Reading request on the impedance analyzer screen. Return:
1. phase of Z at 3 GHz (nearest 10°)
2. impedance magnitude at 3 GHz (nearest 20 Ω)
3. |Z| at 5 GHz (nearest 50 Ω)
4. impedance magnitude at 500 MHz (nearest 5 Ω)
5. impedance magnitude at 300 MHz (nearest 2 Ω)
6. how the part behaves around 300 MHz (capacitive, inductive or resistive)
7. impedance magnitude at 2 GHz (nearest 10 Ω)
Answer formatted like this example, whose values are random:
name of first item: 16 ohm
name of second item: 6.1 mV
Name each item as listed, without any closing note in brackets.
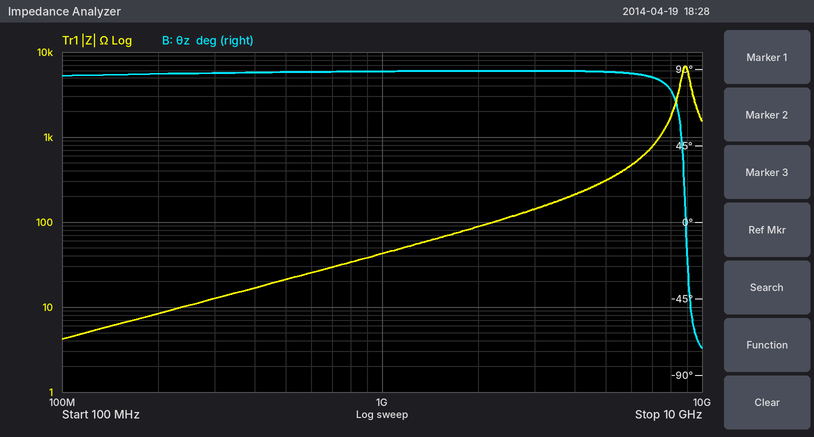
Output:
phase of Z at 3 GHz: 90°
impedance magnitude at 3 GHz: 140 Ω
|Z| at 5 GHz: 300 Ω
impedance magnitude at 500 MHz: 20 Ω
impedance magnitude at 300 MHz: 12 Ω
how the part behaves around 300 MHz: inductive
impedance magnitude at 2 GHz: 90 Ω
